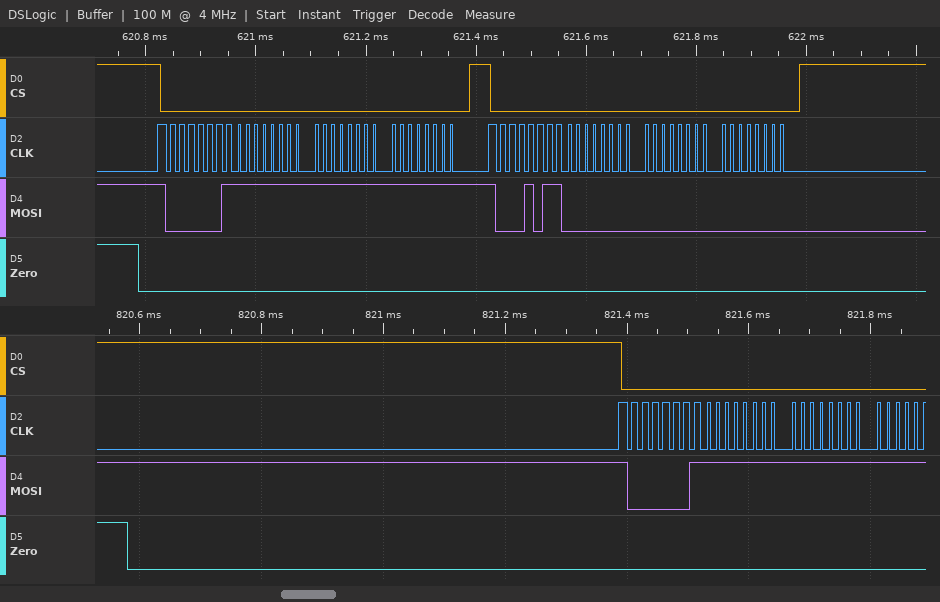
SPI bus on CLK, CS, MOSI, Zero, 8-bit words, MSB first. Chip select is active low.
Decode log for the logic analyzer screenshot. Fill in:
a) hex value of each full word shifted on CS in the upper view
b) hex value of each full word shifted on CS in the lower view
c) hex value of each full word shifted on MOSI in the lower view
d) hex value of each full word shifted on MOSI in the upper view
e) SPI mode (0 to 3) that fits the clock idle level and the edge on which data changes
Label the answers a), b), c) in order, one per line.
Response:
a) 80, 00, 00, 00, 80, 00, 00, 00
b) 80, 00, 00
c) 81, FF, FF
d) 81, FF, FF, FF, 8B, 00, 00, 00
e) 0
